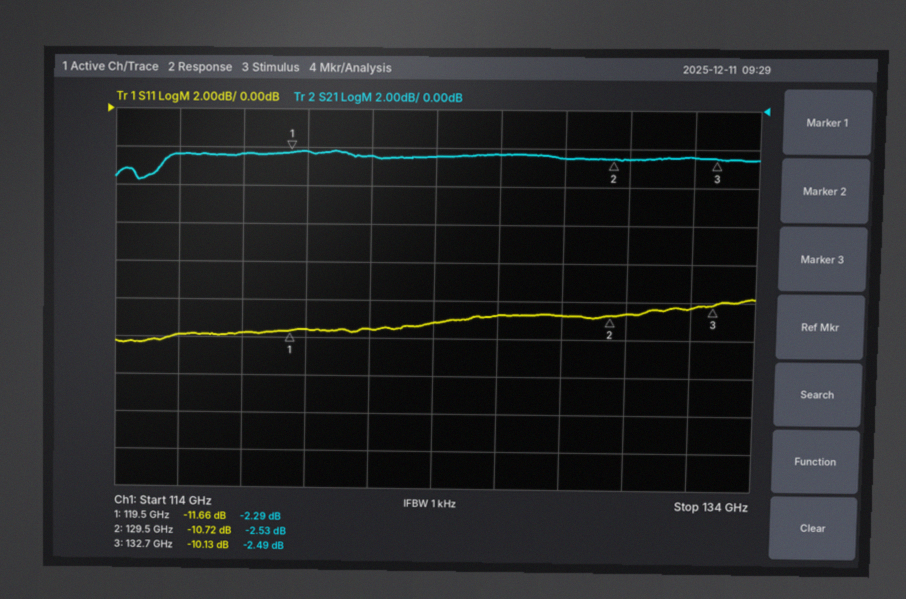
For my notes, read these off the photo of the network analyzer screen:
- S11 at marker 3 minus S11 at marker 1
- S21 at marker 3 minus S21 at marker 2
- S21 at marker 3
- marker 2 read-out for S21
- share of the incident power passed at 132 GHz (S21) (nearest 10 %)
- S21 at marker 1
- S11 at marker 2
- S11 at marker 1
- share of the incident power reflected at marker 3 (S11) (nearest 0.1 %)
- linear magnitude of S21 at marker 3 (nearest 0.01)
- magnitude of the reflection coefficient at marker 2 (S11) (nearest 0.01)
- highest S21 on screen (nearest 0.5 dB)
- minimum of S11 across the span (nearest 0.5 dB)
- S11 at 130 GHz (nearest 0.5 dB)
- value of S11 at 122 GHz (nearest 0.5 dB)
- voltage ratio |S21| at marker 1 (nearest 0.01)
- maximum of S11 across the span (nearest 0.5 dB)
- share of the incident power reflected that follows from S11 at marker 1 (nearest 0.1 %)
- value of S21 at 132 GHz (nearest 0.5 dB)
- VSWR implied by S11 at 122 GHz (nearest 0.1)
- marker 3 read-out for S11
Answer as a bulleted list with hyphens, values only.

- 1.53 dB
- 0.04 dB
- -2.49 dB
- -2.53 dB
- 60 %
- -2.29 dB
- -10.72 dB
- -11.66 dB
- 9.7 %
- 0.75
- 0.29
- -2.0 dB
- -12.5 dB
- -10.5 dB
- -11.5 dB
- 0.77
- -10.0 dB
- 6.8 %
- -2.5 dB
- 1.7
- -10.13 dB
